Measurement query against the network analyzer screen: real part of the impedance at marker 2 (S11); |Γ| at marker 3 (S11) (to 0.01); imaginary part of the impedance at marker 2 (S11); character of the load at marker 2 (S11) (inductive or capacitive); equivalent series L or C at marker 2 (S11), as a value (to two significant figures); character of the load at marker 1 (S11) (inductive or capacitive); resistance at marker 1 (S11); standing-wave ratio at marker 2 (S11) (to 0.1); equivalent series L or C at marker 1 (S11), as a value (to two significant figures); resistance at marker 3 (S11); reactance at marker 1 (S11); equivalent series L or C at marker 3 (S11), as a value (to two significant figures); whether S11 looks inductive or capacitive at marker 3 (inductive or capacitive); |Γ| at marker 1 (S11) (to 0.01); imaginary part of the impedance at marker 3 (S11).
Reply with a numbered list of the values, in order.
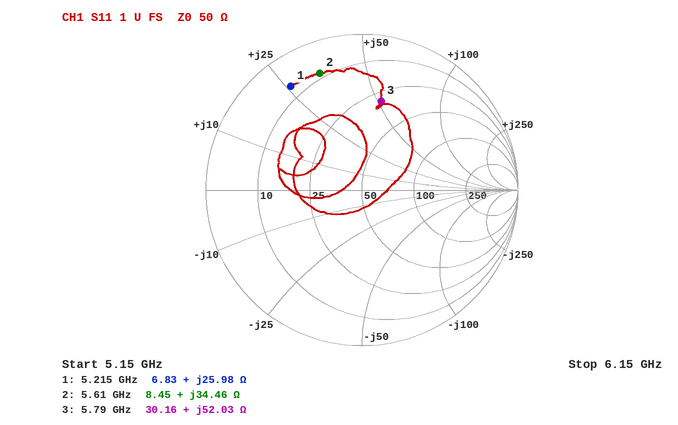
1. 8.45 Ω
2. 0.58
3. +34.46 Ω
4. inductive
5. 980 pH
6. inductive
7. 6.83 Ω
8. 8.8
9. 790 pH
10. 30.16 Ω
11. +25.98 Ω
12. 1.4 nH
13. inductive
14. 0.81
15. +52.03 Ω
